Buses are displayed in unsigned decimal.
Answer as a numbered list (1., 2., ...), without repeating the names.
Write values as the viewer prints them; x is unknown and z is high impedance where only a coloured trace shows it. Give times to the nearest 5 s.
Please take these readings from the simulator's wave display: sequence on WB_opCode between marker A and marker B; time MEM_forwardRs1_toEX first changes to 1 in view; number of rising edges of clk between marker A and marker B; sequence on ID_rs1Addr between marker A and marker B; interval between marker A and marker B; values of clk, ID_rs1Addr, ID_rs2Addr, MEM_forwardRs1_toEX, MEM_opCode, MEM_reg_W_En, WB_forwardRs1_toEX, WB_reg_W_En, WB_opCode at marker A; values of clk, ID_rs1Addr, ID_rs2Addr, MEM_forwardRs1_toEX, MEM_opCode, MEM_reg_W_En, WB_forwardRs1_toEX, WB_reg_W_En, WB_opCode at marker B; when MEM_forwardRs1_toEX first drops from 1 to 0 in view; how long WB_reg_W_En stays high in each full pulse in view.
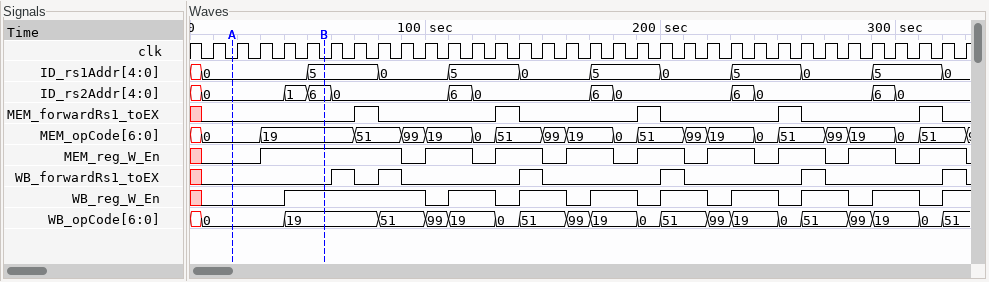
1. 0, 19
2. 70 s
3. 4
4. 0, 5
5. 40 s
6. clk=0, ID_rs1Addr=0, ID_rs2Addr=0, MEM_forwardRs1_toEX=0, MEM_opCode=0, MEM_reg_W_En=0, WB_forwardRs1_toEX=0, WB_reg_W_En=0, WB_opCode=0
7. clk=0, ID_rs1Addr=5, ID_rs2Addr=6, MEM_forwardRs1_toEX=0, MEM_opCode=19, MEM_reg_W_En=1, WB_forwardRs1_toEX=0, WB_reg_W_En=1, WB_opCode=19
8. 80 s
9. 60 s, 20 s, 20 s, 20 s, 20 s, 20 s, 20 s, 20 s
